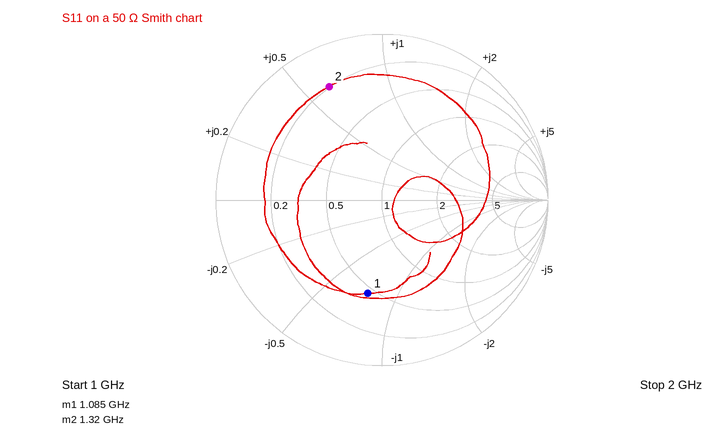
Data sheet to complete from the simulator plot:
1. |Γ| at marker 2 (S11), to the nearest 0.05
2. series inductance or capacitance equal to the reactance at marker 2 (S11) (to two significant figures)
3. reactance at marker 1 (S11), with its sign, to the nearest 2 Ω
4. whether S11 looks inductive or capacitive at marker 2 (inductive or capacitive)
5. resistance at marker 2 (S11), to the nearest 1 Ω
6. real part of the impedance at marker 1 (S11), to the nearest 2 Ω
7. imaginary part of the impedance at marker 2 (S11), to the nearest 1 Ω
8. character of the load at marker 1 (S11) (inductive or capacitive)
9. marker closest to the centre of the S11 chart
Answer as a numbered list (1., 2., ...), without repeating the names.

1. 0.75
2. 3.7 nH
3. -38 Ω
4. inductive
5. 10 Ω
6. 22 Ω
7. +31 Ω
8. capacitive
9. marker 1
